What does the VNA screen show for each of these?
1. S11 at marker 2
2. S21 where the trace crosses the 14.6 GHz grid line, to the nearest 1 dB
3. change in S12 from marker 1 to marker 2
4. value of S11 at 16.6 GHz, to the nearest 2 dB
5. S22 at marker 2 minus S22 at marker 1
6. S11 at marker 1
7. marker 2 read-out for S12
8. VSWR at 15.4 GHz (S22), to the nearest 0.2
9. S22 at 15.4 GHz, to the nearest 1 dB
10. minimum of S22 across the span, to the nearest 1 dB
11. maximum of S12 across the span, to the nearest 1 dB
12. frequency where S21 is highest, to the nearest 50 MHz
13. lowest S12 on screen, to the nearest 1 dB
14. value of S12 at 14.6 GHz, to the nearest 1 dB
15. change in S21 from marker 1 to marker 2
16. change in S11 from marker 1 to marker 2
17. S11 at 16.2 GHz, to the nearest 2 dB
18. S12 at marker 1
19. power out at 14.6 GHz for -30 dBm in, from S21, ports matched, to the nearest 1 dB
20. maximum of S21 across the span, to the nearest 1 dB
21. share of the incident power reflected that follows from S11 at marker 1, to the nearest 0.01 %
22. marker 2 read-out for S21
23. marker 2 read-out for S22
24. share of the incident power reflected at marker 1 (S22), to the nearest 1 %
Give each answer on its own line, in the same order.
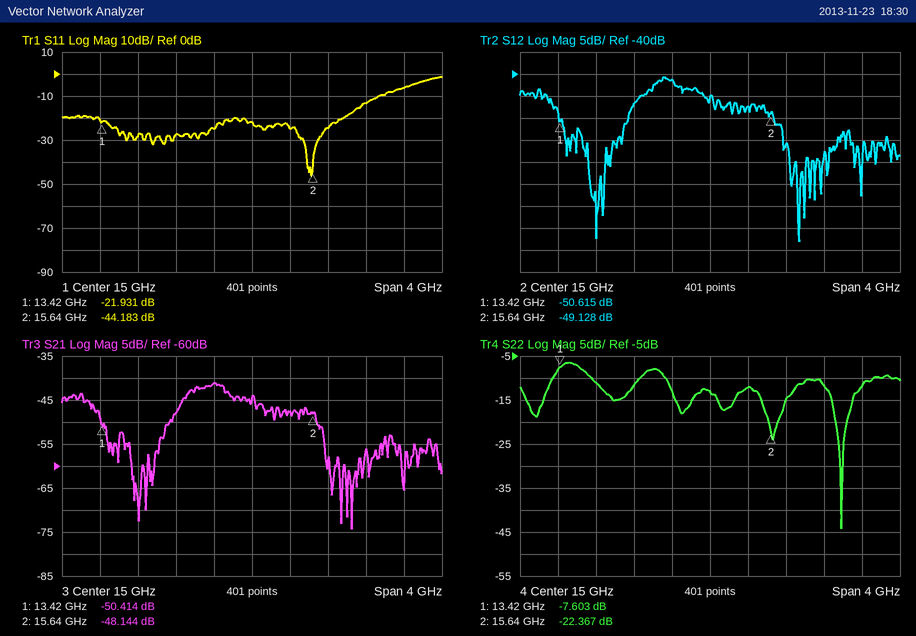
-44.183 dB
-41 dB
1.487 dB
-6 dB
-14.764 dB
-21.931 dB
-49.128 dB
1.6
-12 dB
-44 dB
-41 dB
14.60 GHz
-78 dB
-41 dB
2.270 dB
-22.252 dB
-14 dB
-50.615 dB
-71 dBm
-41 dB
0.64 %
-48.144 dB
-22.367 dB
17 %
